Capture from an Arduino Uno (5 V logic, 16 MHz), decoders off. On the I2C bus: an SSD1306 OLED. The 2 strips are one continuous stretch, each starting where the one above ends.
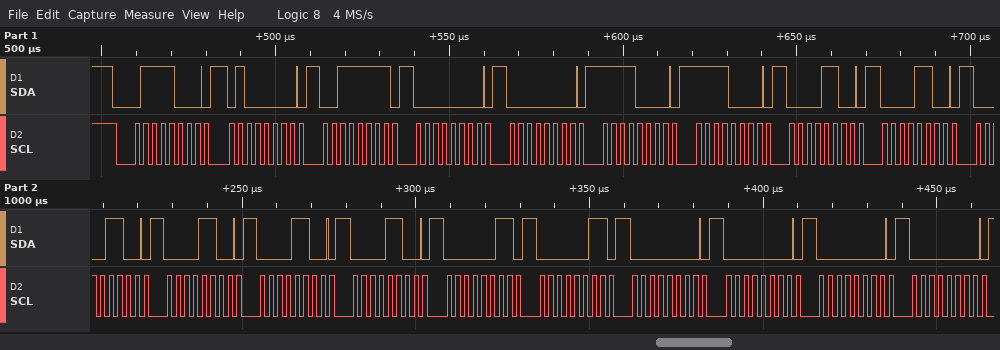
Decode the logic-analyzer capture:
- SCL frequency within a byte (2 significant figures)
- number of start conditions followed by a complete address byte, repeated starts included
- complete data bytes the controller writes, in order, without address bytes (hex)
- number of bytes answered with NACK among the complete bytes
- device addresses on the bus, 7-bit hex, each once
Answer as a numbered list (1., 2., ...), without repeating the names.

1. 400 kHz
2. 1
3. 40 3F 00 00 F0 F0 0C 0C 0C 0C 0C 0C 03 03 00 00 00 00
4. 0
5. 0x3C
